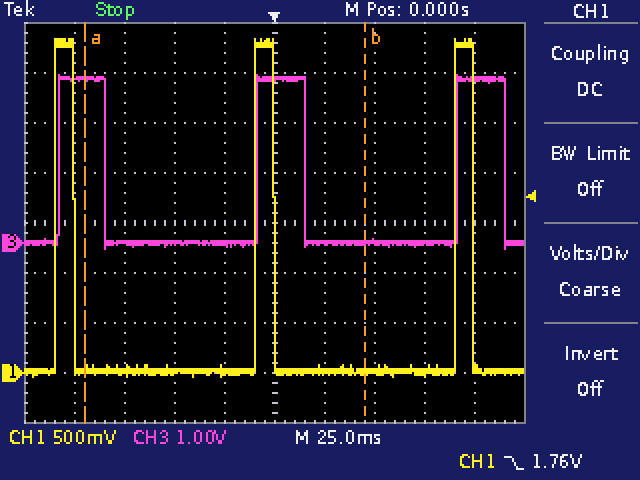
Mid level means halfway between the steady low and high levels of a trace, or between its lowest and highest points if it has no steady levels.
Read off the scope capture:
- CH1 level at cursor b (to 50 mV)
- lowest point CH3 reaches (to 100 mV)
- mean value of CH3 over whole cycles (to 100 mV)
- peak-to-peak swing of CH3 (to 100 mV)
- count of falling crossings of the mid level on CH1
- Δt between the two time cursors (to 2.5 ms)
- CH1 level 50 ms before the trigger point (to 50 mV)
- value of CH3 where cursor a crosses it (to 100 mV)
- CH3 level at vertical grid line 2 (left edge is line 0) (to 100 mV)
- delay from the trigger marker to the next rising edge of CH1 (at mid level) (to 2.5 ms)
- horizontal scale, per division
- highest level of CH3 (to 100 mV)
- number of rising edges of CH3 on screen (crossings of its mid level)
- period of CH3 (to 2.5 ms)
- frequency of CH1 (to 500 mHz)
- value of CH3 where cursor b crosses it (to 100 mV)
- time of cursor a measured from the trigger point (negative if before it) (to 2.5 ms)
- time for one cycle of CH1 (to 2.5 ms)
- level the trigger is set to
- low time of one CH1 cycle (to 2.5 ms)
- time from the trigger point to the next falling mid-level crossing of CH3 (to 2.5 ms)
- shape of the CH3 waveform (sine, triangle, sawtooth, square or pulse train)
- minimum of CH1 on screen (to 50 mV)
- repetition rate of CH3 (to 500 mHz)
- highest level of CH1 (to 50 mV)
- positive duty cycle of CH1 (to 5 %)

0 mV
-100 mV
800 mV
3.5 V
3
140.0 ms
0 mV
3.3 V
0.0 V
90.0 ms
25 ms
3.4 V
3
100.0 ms
10.0 Hz
0.0 V
-95.0 ms
100.0 ms
1.76 V
90.0 ms
15.0 ms
pulse train
-50 mV
10.0 Hz
3.35 V
10 %
